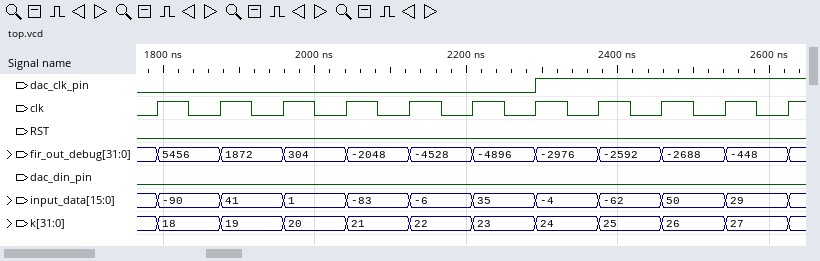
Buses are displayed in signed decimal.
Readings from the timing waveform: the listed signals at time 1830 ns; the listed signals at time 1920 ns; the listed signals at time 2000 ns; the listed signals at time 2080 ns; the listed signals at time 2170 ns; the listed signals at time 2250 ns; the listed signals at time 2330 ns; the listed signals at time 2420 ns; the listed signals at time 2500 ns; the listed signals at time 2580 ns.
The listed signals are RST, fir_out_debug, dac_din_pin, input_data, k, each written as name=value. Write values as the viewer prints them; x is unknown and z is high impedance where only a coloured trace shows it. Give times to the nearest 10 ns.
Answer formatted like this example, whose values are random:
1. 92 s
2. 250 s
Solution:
1. RST=0, fir_out_debug=5456, dac_din_pin=0, input_data=-90, k=18
2. RST=0, fir_out_debug=1872, dac_din_pin=0, input_data=41, k=19
3. RST=0, fir_out_debug=304, dac_din_pin=0, input_data=1, k=20
4. RST=0, fir_out_debug=-2048, dac_din_pin=0, input_data=-83, k=21
5. RST=0, fir_out_debug=-4528, dac_din_pin=0, input_data=-6, k=22
6. RST=0, fir_out_debug=-4896, dac_din_pin=0, input_data=35, k=23
7. RST=0, fir_out_debug=-2976, dac_din_pin=0, input_data=-4, k=24
8. RST=0, fir_out_debug=-2592, dac_din_pin=0, input_data=-62, k=25
9. RST=0, fir_out_debug=-2688, dac_din_pin=0, input_data=50, k=26
10. RST=0, fir_out_debug=-448, dac_din_pin=0, input_data=29, k=27
